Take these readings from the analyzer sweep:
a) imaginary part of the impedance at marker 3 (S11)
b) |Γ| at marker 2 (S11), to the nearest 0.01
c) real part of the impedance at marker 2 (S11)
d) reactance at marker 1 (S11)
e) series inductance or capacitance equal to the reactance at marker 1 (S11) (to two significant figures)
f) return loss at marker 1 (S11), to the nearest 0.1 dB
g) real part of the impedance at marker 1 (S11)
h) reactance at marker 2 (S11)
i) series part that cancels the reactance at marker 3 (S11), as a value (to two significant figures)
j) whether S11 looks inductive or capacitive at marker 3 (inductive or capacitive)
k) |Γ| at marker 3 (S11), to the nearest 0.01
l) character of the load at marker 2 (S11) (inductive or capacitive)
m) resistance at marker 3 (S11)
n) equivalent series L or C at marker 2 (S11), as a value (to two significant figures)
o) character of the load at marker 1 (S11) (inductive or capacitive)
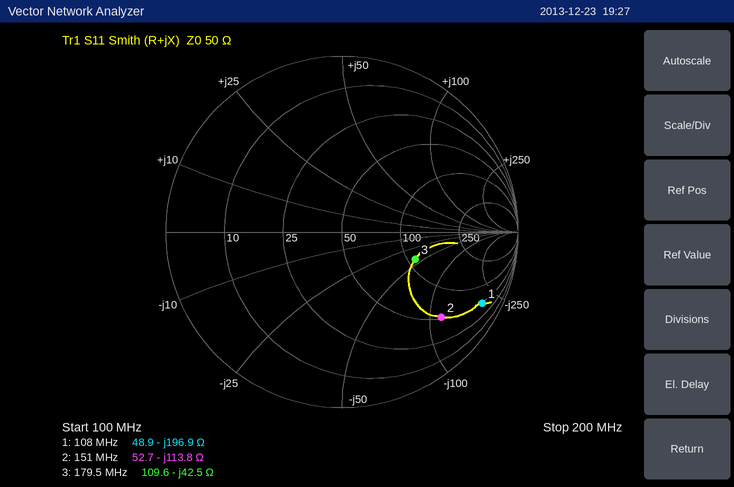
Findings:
-42.5 Ω
0.74
52.7 Ω
-196.9 Ω
7.5 pF
1.0 dB
48.9 Ω
-113.8 Ω
38 nH
capacitive
0.44
capacitive
109.6 Ω
9.3 pF
capacitive
